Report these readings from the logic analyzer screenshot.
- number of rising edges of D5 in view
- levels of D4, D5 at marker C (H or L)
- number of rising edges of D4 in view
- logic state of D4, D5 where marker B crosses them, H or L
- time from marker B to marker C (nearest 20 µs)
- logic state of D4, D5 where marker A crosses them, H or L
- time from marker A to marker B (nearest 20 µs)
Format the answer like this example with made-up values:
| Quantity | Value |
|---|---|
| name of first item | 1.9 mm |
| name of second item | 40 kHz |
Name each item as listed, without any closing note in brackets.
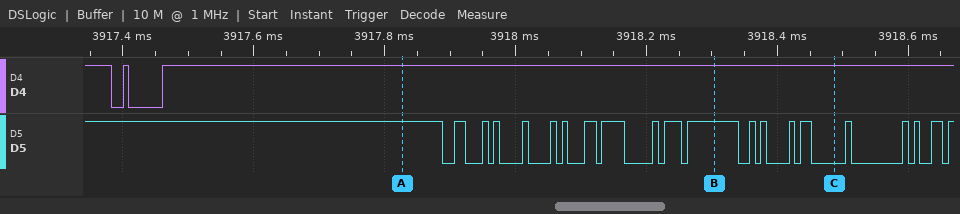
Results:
| Quantity | Value |
|---|---|
| number of rising edges of D5 in view | 20 |
| levels of D4, D5 at marker C | D4=H, D5=L |
| number of rising edges of D4 in view | 2 |
| logic state of D4, D5 where marker B crosses them, H or L | D4=H, D5=H |
| time from marker B to marker C | 180 µs |
| logic state of D4, D5 where marker A crosses them, H or L | D4=H, D5=H |
| time from marker A to marker B | 480 µs |
